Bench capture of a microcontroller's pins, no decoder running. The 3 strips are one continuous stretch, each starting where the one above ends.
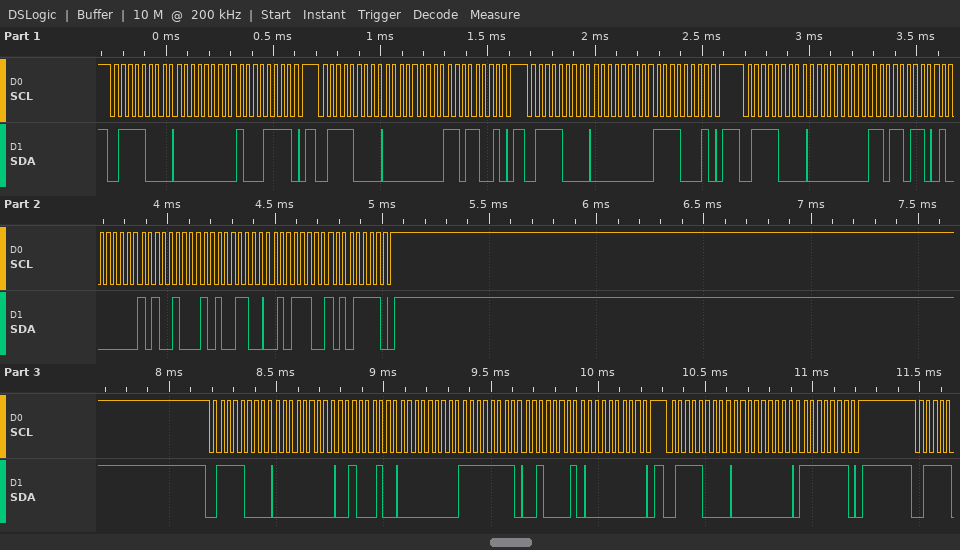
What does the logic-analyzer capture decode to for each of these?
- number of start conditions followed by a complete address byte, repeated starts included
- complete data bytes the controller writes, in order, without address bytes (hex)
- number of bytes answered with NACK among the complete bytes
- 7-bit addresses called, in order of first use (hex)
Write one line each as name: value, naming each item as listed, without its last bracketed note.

number of start conditions followed by a complete address byte, repeated starts included: 6
complete data bytes the controller writes, in order, without address bytes: 00 8F 00 D9 00 F1 00 DB 40 A4 A6 2E AF 00 22 00 FF 21 00 00 7F
number of bytes answered with NACK among the complete bytes: 0
7-bit addresses called, in order of first use: 0x3C
